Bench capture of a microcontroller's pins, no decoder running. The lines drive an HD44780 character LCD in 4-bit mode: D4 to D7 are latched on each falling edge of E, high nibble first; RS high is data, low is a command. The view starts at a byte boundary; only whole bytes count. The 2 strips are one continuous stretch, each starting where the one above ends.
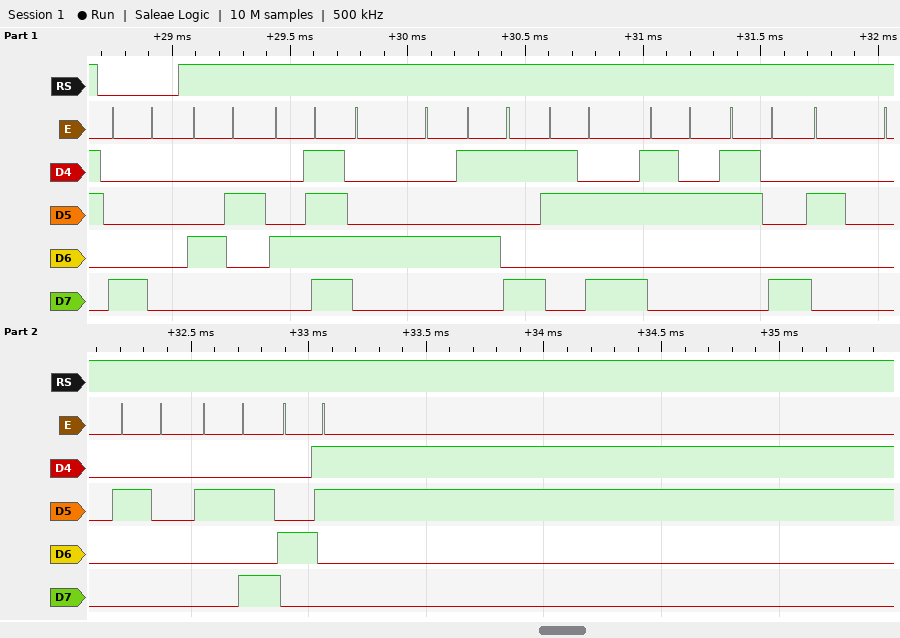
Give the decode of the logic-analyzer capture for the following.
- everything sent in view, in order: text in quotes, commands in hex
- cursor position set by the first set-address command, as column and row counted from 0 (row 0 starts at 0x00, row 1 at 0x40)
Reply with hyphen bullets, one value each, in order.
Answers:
- 0x80 "BODY:28  *C"
- column 0, row 0
